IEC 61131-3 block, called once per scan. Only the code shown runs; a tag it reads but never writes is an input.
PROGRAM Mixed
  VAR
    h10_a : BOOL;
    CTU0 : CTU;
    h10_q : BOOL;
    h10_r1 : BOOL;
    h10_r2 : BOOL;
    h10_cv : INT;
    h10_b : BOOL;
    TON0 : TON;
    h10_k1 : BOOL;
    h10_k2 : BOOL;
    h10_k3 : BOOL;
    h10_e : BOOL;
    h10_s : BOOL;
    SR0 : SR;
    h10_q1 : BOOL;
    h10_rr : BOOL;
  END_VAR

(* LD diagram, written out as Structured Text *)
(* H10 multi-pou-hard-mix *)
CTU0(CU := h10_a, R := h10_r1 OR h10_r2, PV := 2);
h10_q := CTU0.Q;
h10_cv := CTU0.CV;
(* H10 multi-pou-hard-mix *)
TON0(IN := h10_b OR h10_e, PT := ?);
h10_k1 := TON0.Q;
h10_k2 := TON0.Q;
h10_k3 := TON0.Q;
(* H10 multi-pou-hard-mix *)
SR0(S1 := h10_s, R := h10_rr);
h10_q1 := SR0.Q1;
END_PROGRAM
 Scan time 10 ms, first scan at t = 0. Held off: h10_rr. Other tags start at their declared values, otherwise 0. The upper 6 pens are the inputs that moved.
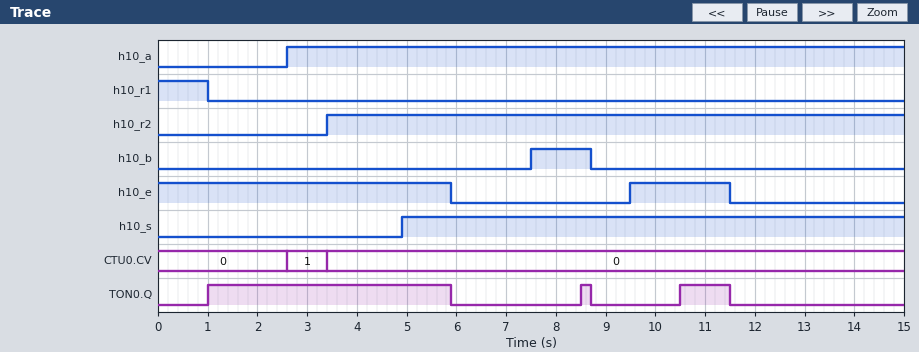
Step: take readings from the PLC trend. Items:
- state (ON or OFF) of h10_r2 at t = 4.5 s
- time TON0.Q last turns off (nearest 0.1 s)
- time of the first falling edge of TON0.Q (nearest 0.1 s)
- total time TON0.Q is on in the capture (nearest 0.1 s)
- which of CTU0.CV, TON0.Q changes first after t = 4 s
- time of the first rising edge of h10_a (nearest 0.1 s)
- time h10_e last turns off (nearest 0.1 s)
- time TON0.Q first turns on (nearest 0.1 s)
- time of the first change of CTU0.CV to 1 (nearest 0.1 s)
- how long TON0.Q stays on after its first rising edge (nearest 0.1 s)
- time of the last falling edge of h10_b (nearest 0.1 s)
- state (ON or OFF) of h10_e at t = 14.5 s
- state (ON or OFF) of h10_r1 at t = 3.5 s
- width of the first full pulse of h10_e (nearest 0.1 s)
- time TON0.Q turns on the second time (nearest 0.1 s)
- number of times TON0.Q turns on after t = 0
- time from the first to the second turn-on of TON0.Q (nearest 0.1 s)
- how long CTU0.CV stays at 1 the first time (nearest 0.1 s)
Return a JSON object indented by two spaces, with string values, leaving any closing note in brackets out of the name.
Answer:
{
  "state (ON or OFF) of h10_r2 at t = 4.5 s": "ON",
  "time TON0.Q last turns off": "11.5 s",
  "time of the first falling edge of TON0.Q": "5.9 s",
  "total time TON0.Q is on in the capture": "6.1 s",
  "which of CTU0.CV, TON0.Q changes first after t = 4 s": "TON0.Q",
  "time of the first rising edge of h10_a": "2.6 s",
  "time h10_e last turns off": "11.5 s",
  "time TON0.Q first turns on": "1.0 s",
  "time of the first change of CTU0.CV to 1": "2.6 s",
  "how long TON0.Q stays on after its first rising edge": "4.9 s",
  "time of the last falling edge of h10_b": "8.7 s",
  "state (ON or OFF) of h10_e at t = 14.5 s": "OFF",
  "state (ON or OFF) of h10_r1 at t = 3.5 s": "OFF",
  "width of the first full pulse of h10_e": "2.0 s",
  "time TON0.Q turns on the second time": "8.5 s",
  "number of times TON0.Q turns on after t = 0": "3",
  "time from the first to the second turn-on of TON0.Q": "7.5 s",
  "how long CTU0.CV stays at 1 the first time": "0.8 s"
}
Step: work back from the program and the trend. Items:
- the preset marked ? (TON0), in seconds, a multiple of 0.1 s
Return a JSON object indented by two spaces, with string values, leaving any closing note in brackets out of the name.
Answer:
{
  "the preset marked ? (TON0), in seconds, a multiple of 0.1 s": "1.0 s"
}
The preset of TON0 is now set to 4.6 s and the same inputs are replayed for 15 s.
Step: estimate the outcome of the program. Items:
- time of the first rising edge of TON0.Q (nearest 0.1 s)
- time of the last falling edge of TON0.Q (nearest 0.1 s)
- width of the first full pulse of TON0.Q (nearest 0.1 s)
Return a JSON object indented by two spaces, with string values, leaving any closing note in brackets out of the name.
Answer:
{
  "time of the first rising edge of TON0.Q": "4.6 s",
  "time of the last falling edge of TON0.Q": "5.9 s",
  "width of the first full pulse of TON0.Q": "1.3 s"
}
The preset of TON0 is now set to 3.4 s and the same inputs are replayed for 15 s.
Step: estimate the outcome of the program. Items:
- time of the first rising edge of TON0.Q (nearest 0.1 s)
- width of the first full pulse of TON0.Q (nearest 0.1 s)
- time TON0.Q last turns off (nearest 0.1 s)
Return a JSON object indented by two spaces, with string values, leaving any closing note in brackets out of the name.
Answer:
{
  "time of the first rising edge of TON0.Q": "3.4 s",
  "width of the first full pulse of TON0.Q": "2.5 s",
  "time TON0.Q last turns off": "5.9 s"
}
